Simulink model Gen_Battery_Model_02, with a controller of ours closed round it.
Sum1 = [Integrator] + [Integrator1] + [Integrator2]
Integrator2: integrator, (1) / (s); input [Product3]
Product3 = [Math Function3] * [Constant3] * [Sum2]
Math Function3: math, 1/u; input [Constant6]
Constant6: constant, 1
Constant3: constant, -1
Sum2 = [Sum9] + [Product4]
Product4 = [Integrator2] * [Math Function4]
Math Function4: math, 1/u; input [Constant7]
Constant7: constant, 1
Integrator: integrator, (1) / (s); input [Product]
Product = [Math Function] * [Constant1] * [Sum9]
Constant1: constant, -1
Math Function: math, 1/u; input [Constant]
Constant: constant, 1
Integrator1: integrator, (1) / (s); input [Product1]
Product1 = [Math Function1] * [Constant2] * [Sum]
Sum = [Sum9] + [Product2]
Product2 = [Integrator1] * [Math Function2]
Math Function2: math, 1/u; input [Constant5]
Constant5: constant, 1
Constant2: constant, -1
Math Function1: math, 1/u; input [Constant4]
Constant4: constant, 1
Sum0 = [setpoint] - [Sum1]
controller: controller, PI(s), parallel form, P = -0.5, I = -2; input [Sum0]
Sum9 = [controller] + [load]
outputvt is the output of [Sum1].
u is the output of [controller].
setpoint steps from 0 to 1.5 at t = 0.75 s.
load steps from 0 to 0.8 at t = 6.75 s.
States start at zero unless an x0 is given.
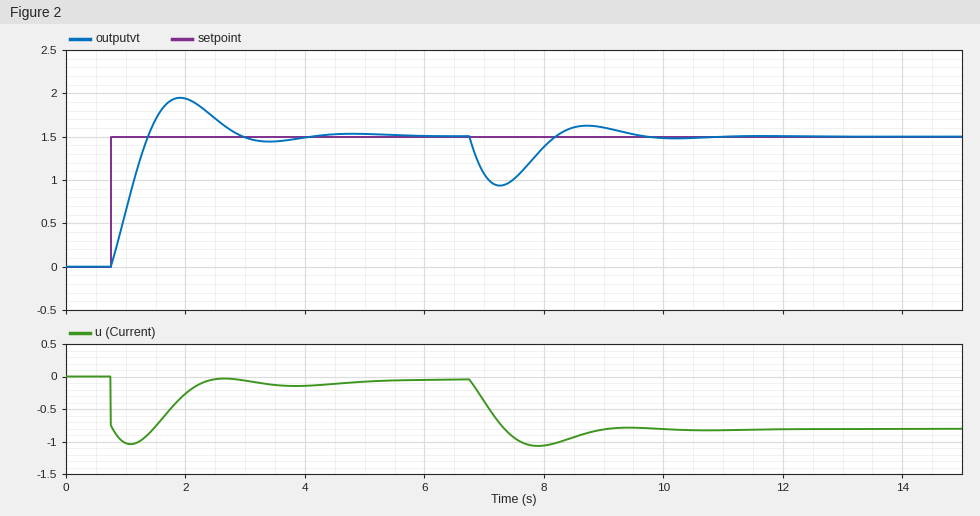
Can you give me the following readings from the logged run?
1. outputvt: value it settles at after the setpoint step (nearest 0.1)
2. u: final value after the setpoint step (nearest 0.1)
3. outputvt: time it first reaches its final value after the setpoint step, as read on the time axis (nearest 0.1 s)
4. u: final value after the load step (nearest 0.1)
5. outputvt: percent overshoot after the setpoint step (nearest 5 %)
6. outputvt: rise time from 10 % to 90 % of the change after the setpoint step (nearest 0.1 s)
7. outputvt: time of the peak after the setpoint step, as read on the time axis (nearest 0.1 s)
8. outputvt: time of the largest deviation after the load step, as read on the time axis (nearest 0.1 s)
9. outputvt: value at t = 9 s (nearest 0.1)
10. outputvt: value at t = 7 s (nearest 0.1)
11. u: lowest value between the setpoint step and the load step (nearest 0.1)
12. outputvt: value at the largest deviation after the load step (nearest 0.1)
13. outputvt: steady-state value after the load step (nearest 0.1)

1.5
0.0
1.4 s
-0.8
30 %
0.5 s
1.9 s
7.3 s
1.6
1.1
-1.0
0.9
1.5
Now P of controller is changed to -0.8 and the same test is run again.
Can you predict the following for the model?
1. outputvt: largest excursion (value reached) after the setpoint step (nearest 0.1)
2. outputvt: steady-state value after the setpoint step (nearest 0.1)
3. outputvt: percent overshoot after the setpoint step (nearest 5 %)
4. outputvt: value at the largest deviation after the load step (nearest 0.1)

1.8
1.5
20 %
1.0
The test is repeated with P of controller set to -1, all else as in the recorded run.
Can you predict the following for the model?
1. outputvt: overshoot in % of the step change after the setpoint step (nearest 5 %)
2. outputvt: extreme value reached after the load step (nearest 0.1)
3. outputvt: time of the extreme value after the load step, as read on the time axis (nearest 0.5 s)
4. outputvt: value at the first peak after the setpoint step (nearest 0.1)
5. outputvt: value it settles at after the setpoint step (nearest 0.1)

15 %
1.1
7.0 s
1.7
1.5
